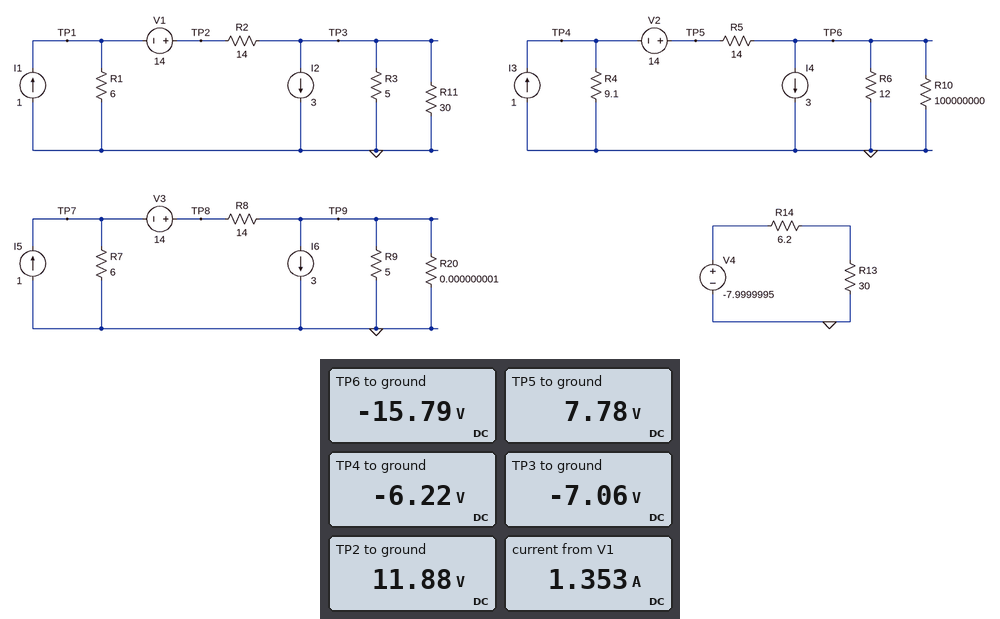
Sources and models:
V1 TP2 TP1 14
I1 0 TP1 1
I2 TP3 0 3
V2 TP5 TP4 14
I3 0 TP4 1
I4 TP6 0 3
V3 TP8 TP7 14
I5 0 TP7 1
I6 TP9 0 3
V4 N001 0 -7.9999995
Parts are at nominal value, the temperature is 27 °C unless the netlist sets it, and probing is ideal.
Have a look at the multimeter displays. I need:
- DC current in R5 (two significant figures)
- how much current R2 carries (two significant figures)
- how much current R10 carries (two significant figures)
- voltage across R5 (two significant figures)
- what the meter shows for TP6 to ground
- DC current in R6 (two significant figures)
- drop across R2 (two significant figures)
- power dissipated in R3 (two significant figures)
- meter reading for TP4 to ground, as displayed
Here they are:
1.7 A
1.4 A
160 nA
24 V
-15.79 V
1.3 A
19 V
10 W
-6.22 V
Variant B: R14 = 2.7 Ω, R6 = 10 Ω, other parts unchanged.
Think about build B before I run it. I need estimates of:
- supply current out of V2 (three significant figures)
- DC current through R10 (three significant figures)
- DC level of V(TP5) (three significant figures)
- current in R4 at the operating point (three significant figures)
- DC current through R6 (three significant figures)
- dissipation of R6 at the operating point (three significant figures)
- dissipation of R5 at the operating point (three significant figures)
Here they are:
1.60 A
140 nA
8.50 V
604 mA
1.40 A
19.5 W
36.0 W
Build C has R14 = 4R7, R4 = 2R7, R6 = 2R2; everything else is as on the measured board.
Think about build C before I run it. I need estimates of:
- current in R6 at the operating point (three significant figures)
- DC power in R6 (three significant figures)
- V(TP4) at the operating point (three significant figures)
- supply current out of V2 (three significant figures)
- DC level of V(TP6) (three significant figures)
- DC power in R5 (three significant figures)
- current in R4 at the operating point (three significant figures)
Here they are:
1.77 A
6.87 W
-629 mV
1.23 A
-3.89 V
21.3 W
233 mA
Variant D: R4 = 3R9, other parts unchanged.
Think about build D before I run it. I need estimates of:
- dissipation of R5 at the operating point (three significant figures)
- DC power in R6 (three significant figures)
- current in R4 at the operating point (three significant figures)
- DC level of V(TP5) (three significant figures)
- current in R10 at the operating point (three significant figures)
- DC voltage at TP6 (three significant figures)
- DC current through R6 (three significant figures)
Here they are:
45.5 W
17.2 W
803 mA
10.9 V
144 nA
-14.4 V
1.20 A
